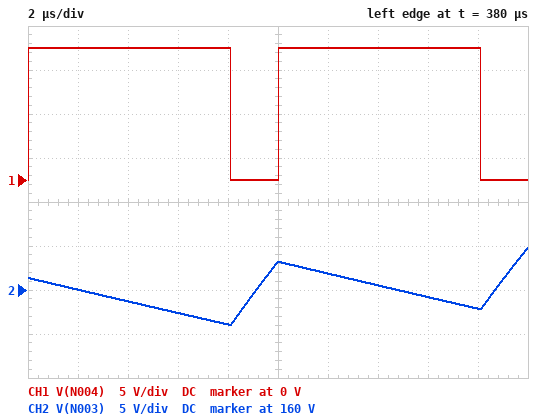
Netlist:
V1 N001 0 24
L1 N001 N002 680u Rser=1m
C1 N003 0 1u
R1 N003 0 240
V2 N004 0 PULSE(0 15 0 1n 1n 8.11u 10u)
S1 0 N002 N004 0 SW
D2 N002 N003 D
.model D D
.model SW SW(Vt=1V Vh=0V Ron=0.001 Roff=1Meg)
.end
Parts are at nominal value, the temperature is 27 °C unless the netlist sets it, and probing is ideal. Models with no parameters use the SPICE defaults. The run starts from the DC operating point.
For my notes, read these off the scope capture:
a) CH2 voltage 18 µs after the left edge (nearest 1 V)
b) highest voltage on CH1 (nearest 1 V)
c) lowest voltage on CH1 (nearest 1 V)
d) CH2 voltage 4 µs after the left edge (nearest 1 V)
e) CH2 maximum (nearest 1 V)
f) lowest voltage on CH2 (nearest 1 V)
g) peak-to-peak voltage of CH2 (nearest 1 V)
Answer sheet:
158 V
15 V
0 V
159 V
165 V
156 V
9 V
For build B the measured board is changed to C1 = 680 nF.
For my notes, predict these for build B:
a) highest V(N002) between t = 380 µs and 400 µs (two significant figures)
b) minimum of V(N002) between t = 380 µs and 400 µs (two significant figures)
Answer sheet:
160 V
3.3 mV
